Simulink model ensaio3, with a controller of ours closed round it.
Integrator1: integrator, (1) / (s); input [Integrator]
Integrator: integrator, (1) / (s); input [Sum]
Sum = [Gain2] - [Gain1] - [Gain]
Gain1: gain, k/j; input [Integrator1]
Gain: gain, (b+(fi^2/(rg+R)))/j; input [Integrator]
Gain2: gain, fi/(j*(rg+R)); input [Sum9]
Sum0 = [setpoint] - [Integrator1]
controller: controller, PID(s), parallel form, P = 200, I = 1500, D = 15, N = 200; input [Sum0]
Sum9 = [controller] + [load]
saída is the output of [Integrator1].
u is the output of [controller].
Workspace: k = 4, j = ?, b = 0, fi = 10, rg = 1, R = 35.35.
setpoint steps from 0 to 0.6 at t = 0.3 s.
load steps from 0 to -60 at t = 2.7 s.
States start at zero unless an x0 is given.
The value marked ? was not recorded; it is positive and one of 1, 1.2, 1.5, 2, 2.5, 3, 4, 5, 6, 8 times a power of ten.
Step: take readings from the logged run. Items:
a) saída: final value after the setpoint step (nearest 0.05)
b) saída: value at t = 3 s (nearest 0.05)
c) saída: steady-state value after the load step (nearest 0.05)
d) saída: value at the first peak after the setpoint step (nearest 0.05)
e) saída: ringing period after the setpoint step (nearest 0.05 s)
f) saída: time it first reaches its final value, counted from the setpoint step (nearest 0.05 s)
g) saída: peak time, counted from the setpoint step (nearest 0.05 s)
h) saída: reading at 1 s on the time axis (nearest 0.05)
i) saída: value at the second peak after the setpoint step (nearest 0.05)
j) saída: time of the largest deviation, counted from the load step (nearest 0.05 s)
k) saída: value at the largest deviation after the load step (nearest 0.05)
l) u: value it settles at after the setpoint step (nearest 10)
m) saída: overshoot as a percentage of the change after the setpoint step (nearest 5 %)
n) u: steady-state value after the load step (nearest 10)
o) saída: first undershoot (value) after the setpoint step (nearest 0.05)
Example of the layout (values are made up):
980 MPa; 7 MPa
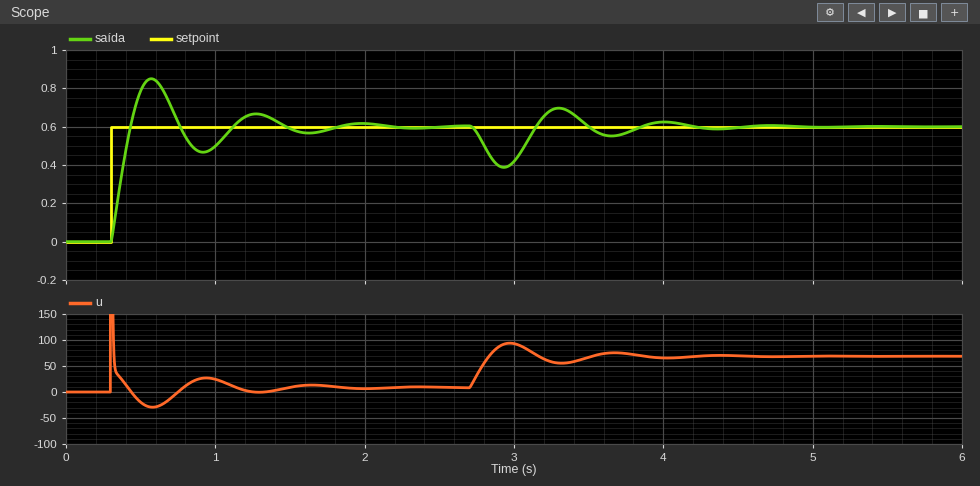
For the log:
0.60; 0.40; 0.60; 0.85; 0.70 s; 0.15 s; 0.25 s; 0.50; 0.65; 0.25 s; 0.40; 10; 40 %; 70; 0.45
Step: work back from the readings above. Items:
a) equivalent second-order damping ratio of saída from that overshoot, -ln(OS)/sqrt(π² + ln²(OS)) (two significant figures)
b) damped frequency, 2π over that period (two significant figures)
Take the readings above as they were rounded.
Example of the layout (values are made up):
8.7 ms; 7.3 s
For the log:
0.28; 9.0 rad/s
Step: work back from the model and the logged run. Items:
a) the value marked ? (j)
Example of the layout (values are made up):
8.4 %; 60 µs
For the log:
0.5
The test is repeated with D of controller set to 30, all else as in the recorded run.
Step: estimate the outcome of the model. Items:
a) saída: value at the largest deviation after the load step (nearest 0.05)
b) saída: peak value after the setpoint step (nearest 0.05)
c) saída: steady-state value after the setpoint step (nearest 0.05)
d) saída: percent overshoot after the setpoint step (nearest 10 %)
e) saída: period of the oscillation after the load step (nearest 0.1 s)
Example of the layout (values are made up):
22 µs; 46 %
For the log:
0.45; 0.70; 0.60; 20 %; 1.0 s
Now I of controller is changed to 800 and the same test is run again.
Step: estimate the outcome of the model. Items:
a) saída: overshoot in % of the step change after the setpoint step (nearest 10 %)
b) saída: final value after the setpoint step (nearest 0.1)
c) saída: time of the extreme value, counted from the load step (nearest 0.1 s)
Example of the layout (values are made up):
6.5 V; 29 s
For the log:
30 %; 0.6; 0.3 s
